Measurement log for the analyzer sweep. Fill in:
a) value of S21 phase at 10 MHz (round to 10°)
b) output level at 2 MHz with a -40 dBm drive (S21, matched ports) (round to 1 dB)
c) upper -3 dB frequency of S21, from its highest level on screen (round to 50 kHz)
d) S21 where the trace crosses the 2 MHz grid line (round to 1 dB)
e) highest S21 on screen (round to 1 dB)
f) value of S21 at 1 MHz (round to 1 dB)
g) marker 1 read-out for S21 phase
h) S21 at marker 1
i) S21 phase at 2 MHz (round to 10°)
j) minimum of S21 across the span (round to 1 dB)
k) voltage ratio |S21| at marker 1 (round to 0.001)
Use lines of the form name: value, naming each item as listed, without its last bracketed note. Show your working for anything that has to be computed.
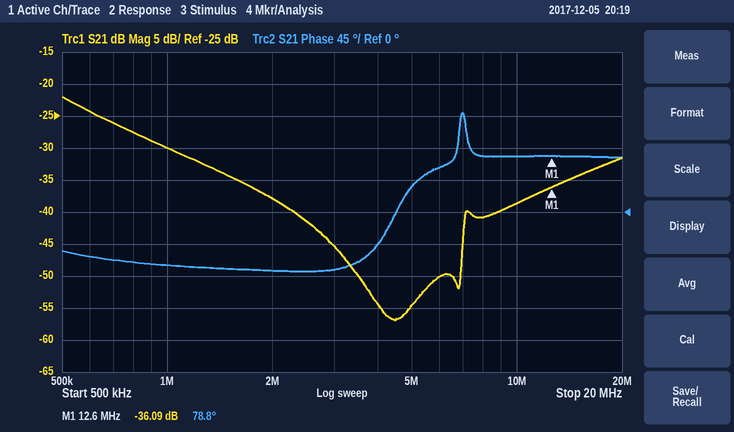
value of S21 phase at 10 MHz: 80°
output level at 2 MHz with a -40 dBm drive (S21, matched ports): -40 dBm + (-38 dB) = -78 dBm
upper -3 dB frequency of S21, from its highest level on screen: 650 kHz
S21 where the trace crosses the 2 MHz grid line: -38 dB
highest S21 on screen: -22 dB
value of S21 at 1 MHz: -30 dB
marker 1 read-out for S21 phase: 78.8°
S21 at marker 1: -36.09 dB
S21 phase at 2 MHz: -80°
minimum of S21 across the span: -57 dB
voltage ratio |S21| at marker 1: 10^(-36.09/20) ≈ 0.016
